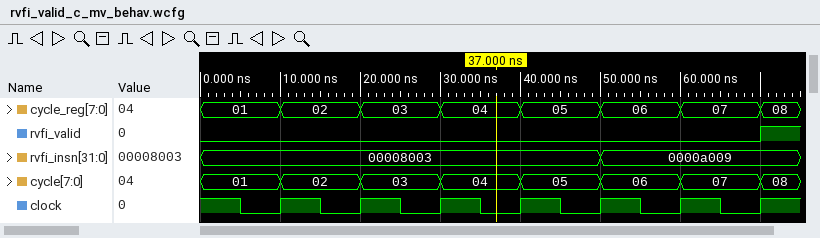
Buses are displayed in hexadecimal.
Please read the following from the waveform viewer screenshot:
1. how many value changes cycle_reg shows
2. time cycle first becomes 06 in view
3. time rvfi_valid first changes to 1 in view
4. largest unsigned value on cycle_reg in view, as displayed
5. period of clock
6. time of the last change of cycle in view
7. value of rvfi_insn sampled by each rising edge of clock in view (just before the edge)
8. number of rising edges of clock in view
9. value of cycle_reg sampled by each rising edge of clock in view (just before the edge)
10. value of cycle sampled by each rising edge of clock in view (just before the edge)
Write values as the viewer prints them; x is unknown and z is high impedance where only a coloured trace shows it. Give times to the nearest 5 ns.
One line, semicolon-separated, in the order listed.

7; 50 ns; 70 ns; 08; 10 ns; 70 ns; 00008003, 00008003, 00008003, 00008003, 00008003, 0000a009, 0000a009; 7; 01, 02, 03, 04, 05, 06, 07; 01, 02, 03, 04, 05, 06, 07
